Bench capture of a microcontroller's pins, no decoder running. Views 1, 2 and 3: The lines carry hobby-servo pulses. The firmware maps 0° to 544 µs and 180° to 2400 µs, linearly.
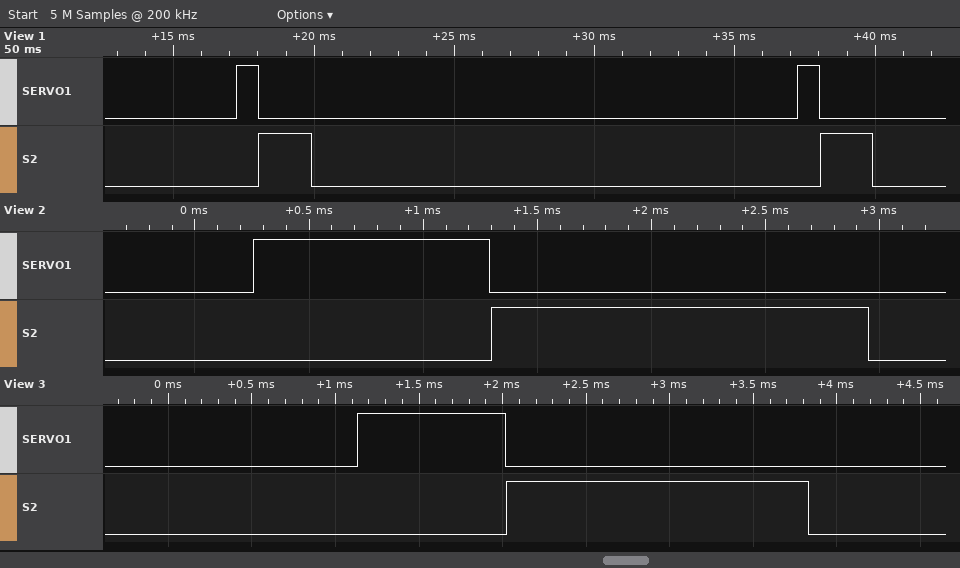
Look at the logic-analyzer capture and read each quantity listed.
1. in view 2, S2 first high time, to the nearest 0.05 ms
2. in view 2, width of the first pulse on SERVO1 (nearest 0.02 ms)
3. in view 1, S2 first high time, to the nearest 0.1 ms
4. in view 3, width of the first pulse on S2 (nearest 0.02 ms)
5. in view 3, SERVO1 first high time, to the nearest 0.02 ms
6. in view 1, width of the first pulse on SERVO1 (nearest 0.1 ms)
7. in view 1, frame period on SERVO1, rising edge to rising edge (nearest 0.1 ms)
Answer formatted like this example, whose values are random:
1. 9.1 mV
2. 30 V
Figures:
1. 1.65 ms
2. 1.04 ms
3. 1.9 ms
4. 1.80 ms
5. 0.88 ms
6. 0.8 ms
7. 20.0 ms
